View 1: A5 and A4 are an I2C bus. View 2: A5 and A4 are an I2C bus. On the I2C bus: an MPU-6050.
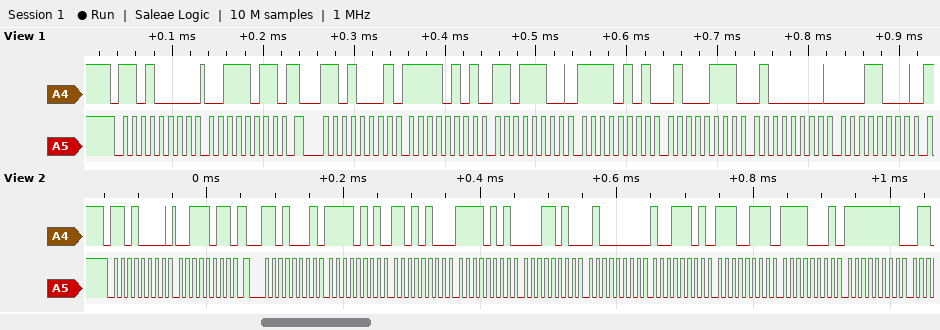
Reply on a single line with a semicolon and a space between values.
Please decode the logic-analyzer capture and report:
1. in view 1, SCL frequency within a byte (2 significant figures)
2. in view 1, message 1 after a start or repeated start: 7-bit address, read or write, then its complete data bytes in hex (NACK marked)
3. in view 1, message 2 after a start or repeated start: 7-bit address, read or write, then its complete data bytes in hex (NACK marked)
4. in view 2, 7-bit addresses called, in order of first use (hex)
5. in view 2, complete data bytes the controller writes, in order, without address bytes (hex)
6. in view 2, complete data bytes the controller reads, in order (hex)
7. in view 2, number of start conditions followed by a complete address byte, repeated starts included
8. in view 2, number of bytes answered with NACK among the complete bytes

100 kHz; 0x68 write: 3B; 0x68 read: F5 DC F5 47 40 18; 0x68; 3B; F5 D4 F5 1A 40 9D E7 F1 FF; 2; 0
